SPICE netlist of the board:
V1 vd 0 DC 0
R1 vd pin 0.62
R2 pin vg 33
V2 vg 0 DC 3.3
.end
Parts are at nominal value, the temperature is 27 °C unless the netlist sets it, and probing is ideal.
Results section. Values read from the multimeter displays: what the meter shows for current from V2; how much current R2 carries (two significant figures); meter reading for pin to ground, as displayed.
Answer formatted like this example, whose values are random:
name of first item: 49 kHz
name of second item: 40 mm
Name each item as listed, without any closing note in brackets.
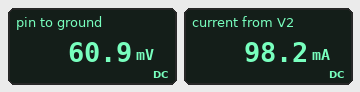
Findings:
what the meter shows for current from V2: 98.2 mA
how much current R2 carries: 98 mA
meter reading for pin to ground, as displayed: 60.9 mV
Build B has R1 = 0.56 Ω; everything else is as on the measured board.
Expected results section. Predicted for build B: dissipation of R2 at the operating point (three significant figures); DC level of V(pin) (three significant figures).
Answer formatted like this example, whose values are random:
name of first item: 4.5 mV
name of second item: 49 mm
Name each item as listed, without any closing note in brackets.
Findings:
dissipation of R2 at the operating point: 319 mW
DC level of V(pin): 55.1 mV
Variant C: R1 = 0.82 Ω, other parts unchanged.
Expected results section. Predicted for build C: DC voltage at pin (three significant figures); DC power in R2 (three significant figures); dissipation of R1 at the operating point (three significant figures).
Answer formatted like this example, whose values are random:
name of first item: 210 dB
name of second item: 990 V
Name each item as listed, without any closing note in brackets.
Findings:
DC voltage at pin: 80.0 mV
DC power in R2: 314 mW
dissipation of R1 at the operating point: 7.81 mW
